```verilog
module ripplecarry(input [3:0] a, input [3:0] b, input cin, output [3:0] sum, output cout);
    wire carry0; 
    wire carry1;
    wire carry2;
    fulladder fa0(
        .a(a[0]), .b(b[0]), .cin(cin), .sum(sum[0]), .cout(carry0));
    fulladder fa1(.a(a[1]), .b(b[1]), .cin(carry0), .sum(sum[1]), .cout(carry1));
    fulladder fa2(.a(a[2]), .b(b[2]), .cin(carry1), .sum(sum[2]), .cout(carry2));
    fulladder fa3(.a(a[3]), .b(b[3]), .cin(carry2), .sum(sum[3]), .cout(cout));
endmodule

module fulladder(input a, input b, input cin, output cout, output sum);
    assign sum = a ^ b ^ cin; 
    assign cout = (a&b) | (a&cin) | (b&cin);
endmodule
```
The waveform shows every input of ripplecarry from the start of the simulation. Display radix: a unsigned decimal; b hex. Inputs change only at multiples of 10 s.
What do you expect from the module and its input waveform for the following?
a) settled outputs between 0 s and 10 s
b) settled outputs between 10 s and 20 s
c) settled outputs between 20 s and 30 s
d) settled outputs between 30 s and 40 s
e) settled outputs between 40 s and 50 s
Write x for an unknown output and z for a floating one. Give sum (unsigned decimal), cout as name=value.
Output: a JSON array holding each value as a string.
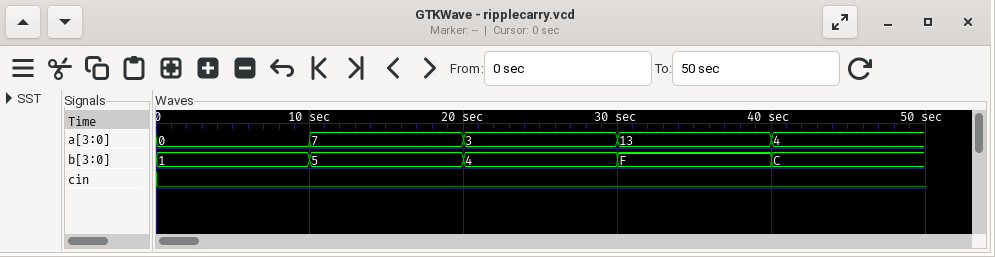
["sum=1, cout=0", "sum=12, cout=0", "sum=7, cout=0", "sum=12, cout=1", "sum=0, cout=1"]
